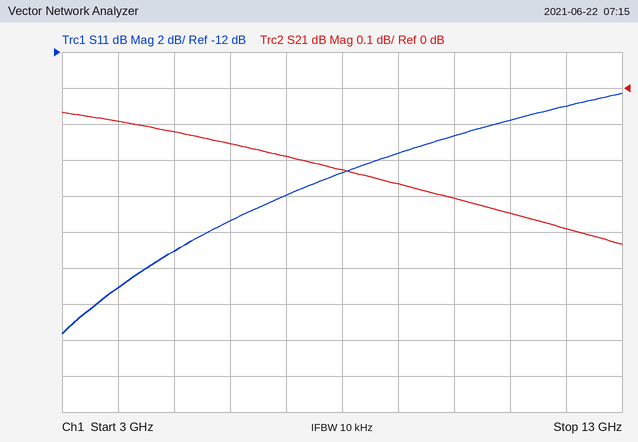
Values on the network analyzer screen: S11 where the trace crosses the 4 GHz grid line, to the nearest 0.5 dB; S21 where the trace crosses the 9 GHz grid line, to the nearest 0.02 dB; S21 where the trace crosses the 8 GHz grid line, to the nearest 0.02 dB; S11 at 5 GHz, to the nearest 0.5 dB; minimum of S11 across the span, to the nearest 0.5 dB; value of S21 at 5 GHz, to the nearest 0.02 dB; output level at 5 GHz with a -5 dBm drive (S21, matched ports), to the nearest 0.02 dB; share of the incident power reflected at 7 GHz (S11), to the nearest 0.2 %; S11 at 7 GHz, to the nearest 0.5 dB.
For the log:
-25.0 dB
-0.26 dB
-0.22 dB
-23.0 dB
-27.5 dB
-0.12 dB
-5.12 dBm
1.0 %
-20.0 dB
